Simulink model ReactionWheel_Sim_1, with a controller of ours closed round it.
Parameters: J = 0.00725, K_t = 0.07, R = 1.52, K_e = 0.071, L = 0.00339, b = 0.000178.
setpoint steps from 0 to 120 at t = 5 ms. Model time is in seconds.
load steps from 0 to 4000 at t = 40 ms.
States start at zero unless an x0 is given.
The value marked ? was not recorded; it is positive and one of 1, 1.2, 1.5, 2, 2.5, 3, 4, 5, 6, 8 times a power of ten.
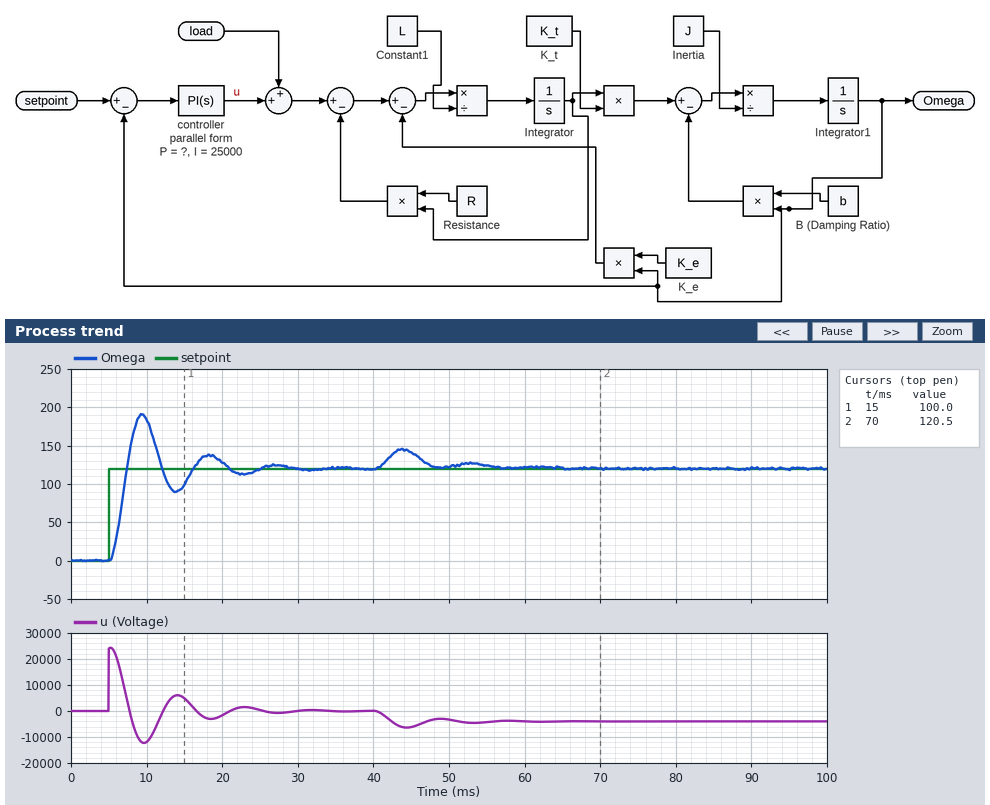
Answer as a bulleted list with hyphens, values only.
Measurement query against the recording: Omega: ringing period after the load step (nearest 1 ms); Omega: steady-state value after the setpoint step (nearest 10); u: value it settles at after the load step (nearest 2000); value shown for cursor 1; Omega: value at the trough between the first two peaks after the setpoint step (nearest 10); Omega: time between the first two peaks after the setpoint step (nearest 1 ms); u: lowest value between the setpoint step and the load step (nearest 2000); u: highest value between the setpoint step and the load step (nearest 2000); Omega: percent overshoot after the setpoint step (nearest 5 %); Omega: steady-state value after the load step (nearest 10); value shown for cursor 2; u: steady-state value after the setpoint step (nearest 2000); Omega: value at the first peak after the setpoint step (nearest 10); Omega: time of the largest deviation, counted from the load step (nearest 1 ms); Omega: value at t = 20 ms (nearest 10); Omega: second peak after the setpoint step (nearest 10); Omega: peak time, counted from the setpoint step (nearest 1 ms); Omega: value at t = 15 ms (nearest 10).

- 9 ms
- 120
- -4000
- 100.0
- 90
- 9 ms
- -12000
- 24000
- 60 %
- 120
- 120.5
- 0
- 190
- 4 ms
- 130
- 140
- 4 ms
- 100
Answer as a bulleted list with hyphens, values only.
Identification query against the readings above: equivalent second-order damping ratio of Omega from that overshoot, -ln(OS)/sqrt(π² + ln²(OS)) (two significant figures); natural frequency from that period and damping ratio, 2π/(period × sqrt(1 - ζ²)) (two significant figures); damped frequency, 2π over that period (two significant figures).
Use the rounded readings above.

- 0.16
- 0.71 rad/ms
- 0.70 rad/ms
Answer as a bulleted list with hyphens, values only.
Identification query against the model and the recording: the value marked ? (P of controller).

- 200
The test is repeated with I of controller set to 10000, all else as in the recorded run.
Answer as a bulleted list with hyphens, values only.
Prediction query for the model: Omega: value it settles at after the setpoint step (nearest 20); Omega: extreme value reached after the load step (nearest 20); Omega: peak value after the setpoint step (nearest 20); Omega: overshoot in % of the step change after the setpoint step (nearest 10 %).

- 120
- 140
- 180
- 50 %
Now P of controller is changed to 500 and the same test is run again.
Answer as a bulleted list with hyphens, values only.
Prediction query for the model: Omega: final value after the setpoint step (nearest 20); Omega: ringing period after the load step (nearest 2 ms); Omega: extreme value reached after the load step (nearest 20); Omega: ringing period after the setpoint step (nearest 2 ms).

- 120
- 6 ms
- 140
- 6 ms
